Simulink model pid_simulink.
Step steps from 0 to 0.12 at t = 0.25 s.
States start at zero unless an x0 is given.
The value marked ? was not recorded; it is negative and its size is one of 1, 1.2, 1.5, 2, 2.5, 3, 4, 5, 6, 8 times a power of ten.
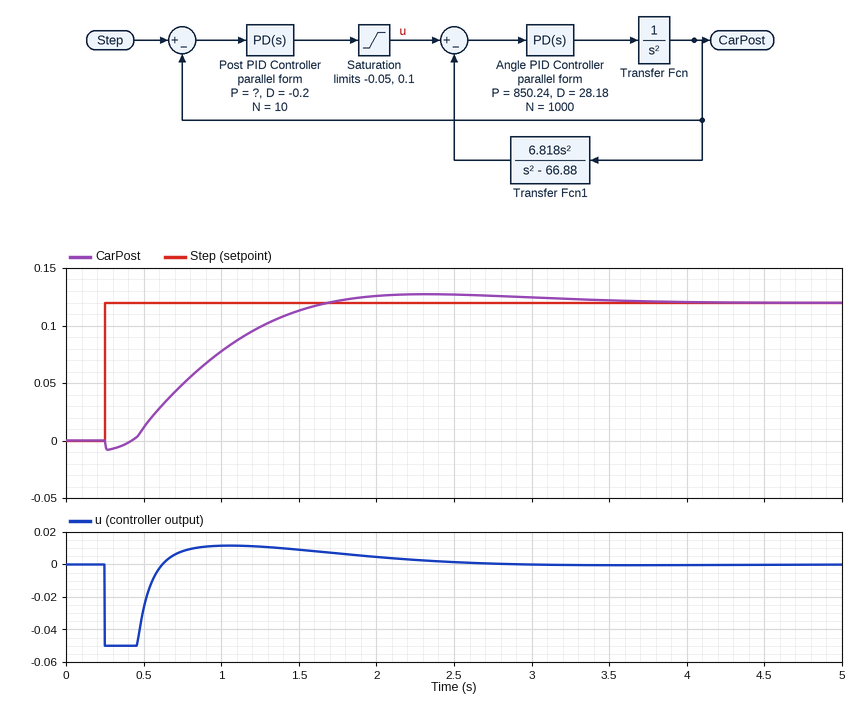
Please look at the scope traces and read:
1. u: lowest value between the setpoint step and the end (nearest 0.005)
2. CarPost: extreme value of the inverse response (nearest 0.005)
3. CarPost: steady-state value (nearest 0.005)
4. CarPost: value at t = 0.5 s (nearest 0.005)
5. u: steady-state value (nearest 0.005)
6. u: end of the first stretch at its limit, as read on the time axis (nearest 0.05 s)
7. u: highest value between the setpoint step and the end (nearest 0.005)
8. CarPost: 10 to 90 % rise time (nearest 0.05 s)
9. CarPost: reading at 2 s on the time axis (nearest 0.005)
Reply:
-0.050
-0.010
0.120
0.010
0.000
0.45 s
0.010
0.90 s
0.125
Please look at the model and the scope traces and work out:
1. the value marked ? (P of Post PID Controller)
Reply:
-0.25
